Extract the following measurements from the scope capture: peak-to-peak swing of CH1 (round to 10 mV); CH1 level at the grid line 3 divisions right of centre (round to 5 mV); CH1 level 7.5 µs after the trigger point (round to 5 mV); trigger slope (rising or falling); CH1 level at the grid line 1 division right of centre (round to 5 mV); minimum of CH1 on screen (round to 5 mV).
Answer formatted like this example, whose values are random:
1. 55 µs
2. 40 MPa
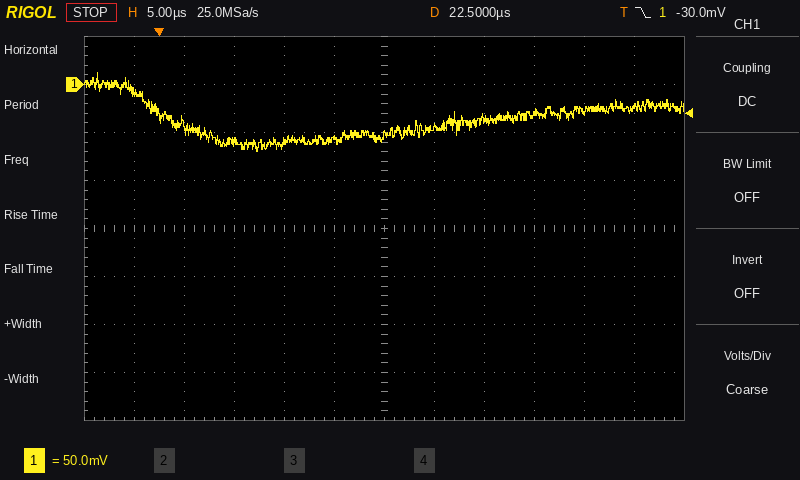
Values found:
1. 80 mV
2. -30 mV
3. -60 mV
4. falling
5. -45 mV
6. -70 mV
